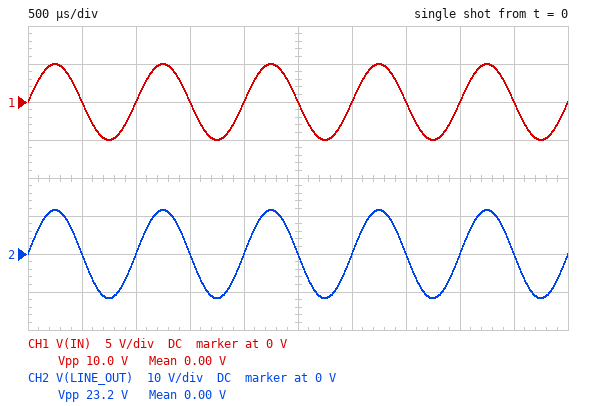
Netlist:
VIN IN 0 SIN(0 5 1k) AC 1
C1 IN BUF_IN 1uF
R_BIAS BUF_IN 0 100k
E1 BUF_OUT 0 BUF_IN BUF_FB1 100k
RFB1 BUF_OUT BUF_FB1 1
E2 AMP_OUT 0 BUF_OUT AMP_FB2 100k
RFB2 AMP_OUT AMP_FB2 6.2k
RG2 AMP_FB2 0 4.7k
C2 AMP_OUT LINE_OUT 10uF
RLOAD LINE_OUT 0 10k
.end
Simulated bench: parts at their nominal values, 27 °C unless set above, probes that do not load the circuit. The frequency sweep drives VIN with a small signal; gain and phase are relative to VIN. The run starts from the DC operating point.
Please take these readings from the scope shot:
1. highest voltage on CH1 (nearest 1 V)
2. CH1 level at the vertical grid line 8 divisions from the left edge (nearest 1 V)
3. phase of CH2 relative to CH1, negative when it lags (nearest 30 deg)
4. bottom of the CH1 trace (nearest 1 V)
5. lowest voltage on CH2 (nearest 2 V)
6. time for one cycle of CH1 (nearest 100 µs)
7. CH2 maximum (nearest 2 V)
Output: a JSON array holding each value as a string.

["5 V", "0 V", "0 deg", "-5 V", "-12 V", "1.0 ms", "12 V"]
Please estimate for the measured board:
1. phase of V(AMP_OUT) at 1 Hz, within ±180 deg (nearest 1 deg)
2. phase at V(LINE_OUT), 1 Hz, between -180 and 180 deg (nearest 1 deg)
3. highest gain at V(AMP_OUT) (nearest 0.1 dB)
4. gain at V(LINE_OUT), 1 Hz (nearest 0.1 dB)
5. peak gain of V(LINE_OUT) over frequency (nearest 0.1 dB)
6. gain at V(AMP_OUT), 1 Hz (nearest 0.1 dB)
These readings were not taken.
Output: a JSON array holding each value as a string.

["58 deg", "116 deg", "7.3 dB", "-3.7 dB", "7.3 dB", "1.8 dB"]
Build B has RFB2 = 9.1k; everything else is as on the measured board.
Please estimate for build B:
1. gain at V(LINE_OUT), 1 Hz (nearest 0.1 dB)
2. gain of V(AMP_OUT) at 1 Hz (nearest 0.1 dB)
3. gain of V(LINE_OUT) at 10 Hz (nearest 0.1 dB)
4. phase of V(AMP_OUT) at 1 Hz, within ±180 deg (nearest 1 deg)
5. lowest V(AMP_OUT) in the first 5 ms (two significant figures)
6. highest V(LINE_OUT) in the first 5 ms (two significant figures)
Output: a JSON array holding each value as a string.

["-1.6 dB", "3.9 dB", "9.1 dB", "58 deg", "-15 V", "15 V"]
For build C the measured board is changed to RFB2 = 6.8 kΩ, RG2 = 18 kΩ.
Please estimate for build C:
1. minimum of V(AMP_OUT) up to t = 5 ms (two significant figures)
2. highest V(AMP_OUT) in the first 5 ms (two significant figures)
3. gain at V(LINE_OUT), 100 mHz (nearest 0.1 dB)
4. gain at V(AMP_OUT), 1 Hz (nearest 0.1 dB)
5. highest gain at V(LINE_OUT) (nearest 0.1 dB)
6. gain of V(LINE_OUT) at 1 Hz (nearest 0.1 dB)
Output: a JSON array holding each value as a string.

["-6.9 V", "6.9 V", "-45.3 dB", "-2.7 dB", "2.8 dB", "-8.2 dB"]
